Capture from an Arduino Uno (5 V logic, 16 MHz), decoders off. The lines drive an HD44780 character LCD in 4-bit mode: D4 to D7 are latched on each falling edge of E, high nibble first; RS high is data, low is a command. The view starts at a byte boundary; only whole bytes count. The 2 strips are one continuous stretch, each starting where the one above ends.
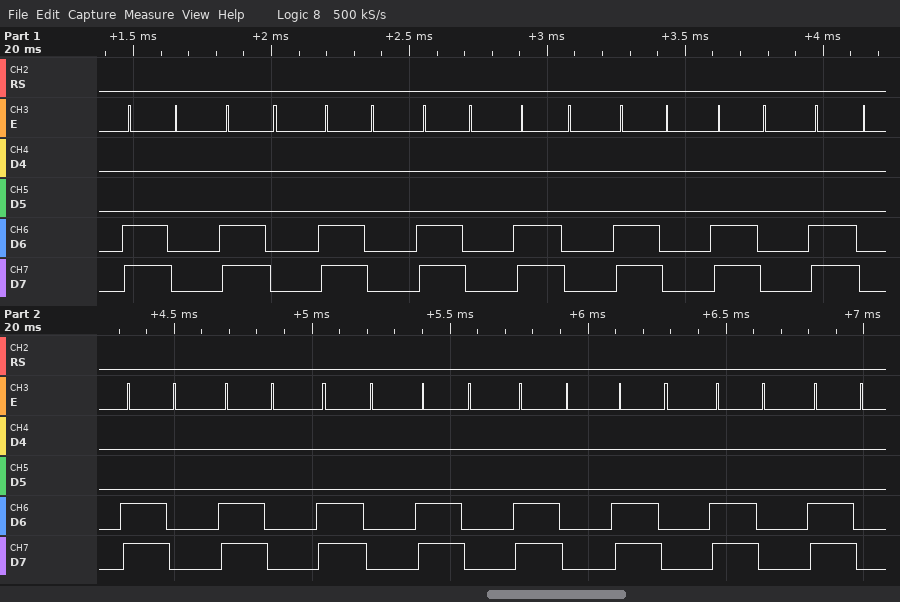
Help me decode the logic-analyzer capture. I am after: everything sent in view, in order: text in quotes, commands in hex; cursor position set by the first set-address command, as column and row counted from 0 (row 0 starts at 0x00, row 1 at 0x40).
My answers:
0xC0 0xC0 0xC0 0xC0 0xC0 0xC0 0xC0 0xC0 0xC0 0xC0 0xC0 0xC0 0xC0 0xC0 0xC0 0xC0
column 0, row 1
